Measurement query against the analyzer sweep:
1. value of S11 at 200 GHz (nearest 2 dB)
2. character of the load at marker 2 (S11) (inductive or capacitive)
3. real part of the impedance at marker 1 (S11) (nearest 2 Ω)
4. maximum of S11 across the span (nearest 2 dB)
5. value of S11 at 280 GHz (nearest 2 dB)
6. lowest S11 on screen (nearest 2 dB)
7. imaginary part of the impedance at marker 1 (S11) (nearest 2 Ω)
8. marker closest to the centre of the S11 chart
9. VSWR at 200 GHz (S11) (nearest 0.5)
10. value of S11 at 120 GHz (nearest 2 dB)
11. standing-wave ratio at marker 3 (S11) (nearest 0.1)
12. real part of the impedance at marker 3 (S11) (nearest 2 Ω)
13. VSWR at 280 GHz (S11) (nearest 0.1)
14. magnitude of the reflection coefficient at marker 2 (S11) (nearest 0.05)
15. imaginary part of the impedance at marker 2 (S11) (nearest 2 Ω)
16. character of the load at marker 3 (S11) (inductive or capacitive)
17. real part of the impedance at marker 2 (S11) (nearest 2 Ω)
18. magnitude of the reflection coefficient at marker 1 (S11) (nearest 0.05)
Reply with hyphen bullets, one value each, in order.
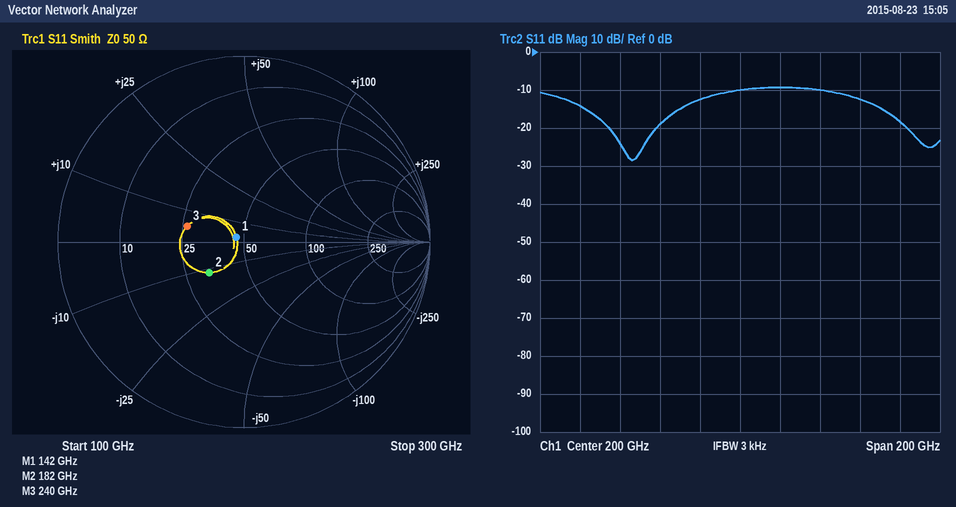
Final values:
- -10 dB
- capacitive
- 46 Ω
- -10 dB
- -18 dB
- -28 dB
- +2 Ω
- marker 1
- 2.0
- -14 dB
- 1.9
- 26 Ω
- 1.3
- 0.25
- -12 Ω
- inductive
- 32 Ω
- 0.05
